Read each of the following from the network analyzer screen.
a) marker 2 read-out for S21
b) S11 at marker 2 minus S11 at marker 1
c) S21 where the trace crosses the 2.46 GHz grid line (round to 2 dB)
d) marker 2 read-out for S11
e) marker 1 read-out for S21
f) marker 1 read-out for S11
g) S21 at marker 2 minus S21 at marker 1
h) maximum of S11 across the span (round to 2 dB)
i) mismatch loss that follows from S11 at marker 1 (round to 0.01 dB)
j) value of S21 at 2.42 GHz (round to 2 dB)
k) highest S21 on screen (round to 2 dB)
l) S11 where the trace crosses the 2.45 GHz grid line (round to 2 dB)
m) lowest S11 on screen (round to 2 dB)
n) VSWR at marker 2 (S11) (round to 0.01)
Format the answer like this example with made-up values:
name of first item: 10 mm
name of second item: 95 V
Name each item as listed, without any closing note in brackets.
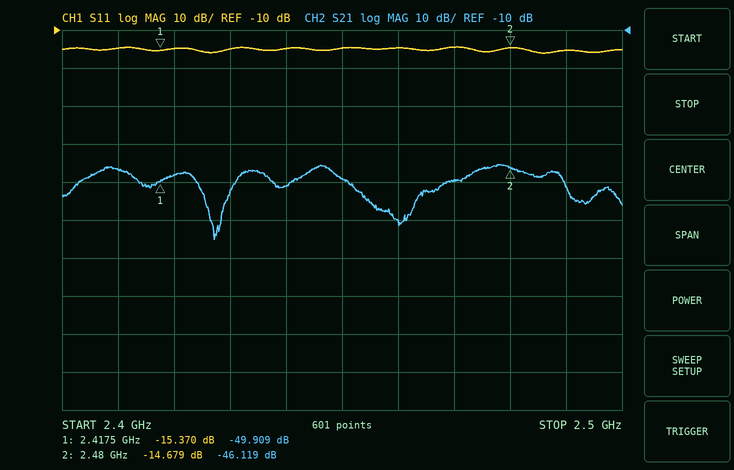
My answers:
marker 2 read-out for S21: -46.119 dB
S11 at marker 2 minus S11 at marker 1: 0.691 dB
S21 where the trace crosses the 2.46 GHz grid line: -60 dB
marker 2 read-out for S11: -14.679 dB
marker 1 read-out for S21: -49.909 dB
marker 1 read-out for S11: -15.370 dB
S21 at marker 2 minus S21 at marker 1: 3.790 dB
maximum of S11 across the span: -14 dB
mismatch loss that follows from S11 at marker 1: 0.13 dB
value of S21 at 2.42 GHz: -48 dB
highest S21 on screen: -46 dB
S11 where the trace crosses the 2.45 GHz grid line: -14 dB
lowest S11 on screen: -16 dB
VSWR at marker 2 (S11): 1.45
